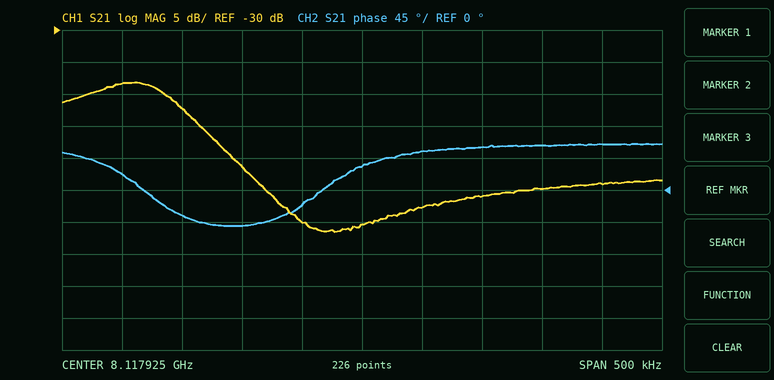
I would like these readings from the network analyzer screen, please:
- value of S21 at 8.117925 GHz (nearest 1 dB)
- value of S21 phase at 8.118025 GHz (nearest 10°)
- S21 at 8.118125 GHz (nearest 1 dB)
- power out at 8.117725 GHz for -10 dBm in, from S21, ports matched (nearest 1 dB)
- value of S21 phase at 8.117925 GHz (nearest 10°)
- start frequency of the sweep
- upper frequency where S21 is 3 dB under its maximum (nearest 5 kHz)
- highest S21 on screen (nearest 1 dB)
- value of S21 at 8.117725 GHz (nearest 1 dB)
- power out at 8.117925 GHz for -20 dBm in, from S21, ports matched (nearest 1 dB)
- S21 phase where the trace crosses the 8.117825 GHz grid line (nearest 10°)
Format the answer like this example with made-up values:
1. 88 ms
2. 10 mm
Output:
1. -60 dB
2. 60°
3. -54 dB
4. -48 dBm
5. 30°
6. 8.117675 GHz
7. 8.117770 GHz
8. -38 dB
9. -38 dB
10. -80 dBm
11. -50°
